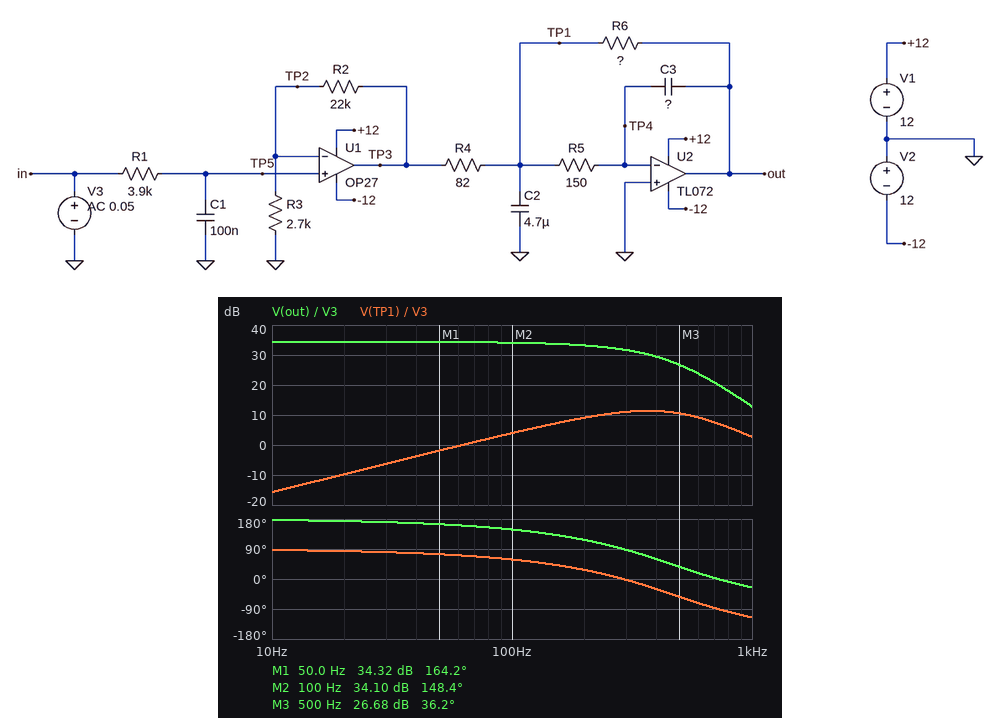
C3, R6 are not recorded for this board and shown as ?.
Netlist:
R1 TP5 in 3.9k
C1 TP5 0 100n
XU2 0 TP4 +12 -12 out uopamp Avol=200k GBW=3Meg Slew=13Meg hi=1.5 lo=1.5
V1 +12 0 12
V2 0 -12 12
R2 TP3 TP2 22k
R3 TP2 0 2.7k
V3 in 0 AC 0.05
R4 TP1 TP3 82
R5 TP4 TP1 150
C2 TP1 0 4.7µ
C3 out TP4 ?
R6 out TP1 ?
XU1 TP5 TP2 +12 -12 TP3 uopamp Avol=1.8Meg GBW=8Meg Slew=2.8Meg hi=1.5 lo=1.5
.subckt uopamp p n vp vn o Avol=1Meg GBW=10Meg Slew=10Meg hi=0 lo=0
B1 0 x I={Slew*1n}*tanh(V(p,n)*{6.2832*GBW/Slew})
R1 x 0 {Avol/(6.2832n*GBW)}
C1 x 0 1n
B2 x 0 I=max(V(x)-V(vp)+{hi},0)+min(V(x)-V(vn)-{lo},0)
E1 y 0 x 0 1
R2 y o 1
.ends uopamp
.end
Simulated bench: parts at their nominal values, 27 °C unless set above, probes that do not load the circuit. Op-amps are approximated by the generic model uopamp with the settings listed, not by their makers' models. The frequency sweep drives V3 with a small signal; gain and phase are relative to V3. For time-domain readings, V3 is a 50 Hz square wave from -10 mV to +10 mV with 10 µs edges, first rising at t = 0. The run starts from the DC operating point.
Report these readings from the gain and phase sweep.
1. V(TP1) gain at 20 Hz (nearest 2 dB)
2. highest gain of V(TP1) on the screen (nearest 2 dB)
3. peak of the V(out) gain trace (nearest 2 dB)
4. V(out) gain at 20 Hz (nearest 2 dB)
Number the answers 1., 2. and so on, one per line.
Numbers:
1. -10 dB
2. 12 dB
3. 34 dB
4. 34 dB
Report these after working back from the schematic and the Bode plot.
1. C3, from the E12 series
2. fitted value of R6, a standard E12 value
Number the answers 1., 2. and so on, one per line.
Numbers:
1. 330 nF
2. 470 Ω
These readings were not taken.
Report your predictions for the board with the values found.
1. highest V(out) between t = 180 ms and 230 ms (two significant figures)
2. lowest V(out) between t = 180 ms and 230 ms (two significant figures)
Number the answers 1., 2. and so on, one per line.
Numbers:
1. 530 mV
2. -530 mV
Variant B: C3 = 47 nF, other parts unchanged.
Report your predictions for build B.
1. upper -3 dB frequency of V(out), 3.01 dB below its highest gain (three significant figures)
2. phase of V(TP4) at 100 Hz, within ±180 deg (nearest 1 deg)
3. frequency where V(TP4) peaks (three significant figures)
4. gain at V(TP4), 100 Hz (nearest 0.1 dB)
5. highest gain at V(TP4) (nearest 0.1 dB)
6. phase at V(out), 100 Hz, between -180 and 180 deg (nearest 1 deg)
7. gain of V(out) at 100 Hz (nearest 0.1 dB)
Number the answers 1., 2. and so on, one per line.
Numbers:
1. 539 Hz
2. 65 deg
3. 1.18 kHz
4. -55.2 dB
5. -38.0 dB
6. 164 deg
7. 34.2 dB
